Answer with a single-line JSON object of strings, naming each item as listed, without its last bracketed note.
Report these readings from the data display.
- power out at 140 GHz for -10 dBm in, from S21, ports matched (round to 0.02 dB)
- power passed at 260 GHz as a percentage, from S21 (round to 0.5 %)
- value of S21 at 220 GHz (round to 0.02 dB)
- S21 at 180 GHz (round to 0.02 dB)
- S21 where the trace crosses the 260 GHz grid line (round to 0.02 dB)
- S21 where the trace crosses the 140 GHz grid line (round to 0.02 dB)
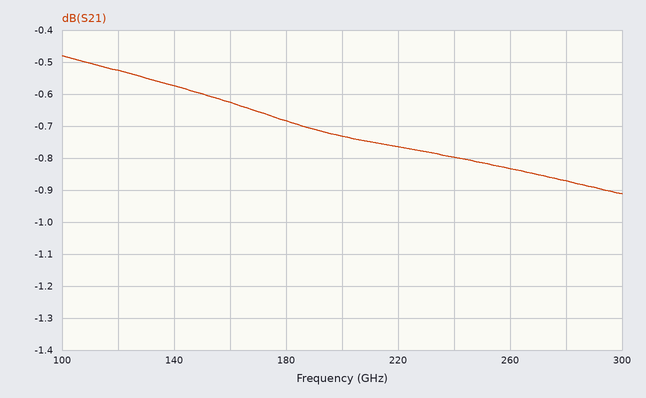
{"power out at 140 GHz for -10 dBm in, from S21, ports matched": "-10.58 dBm", "power passed at 260 GHz as a percentage, from S21": "82.5 %", "value of S21 at 220 GHz": "-0.76 dB", "S21 at 180 GHz": "-0.68 dB", "S21 where the trace crosses the 260 GHz grid line": "-0.84 dB", "S21 where the trace crosses the 140 GHz grid line": "-0.58 dB"}
